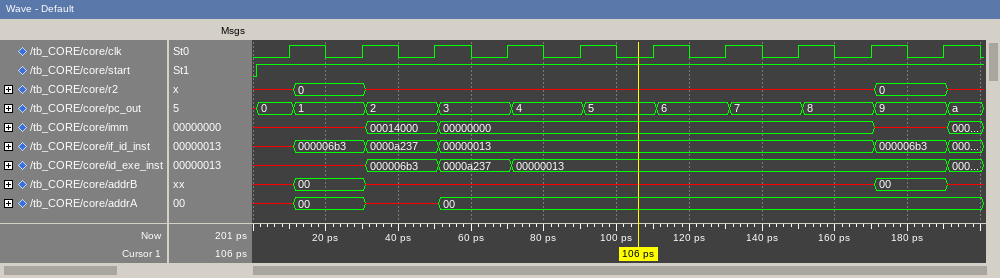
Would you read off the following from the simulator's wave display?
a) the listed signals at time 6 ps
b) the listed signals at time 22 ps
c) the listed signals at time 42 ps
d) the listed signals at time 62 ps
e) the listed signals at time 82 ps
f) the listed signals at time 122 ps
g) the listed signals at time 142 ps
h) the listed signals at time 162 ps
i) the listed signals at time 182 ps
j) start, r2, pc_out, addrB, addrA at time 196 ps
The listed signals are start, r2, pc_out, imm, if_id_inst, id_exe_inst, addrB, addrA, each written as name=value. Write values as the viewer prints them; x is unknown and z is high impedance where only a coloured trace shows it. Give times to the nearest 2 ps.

start=1, r2=x, pc_out=0, imm=x, if_id_inst=x, id_exe_inst=x, addrB=x, addrA=x
start=1, r2=0, pc_out=1, imm=x, if_id_inst=000006b3, id_exe_inst=x, addrB=00, addrA=00
start=1, r2=x, pc_out=2, imm=00014000, if_id_inst=0000a237, id_exe_inst=000006b3, addrB=x, addrA=x
start=1, r2=x, pc_out=3, imm=00000000, if_id_inst=00000013, id_exe_inst=0000a237, addrB=x, addrA=00
start=1, r2=x, pc_out=4, imm=00000000, if_id_inst=00000013, id_exe_inst=00000013, addrB=x, addrA=00
start=1, r2=x, pc_out=6, imm=00000000, if_id_inst=00000013, id_exe_inst=00000013, addrB=x, addrA=00
start=1, r2=x, pc_out=7, imm=00000000, if_id_inst=00000013, id_exe_inst=00000013, addrB=x, addrA=00
start=1, r2=x, pc_out=8, imm=00000000, if_id_inst=00000013, id_exe_inst=00000013, addrB=x, addrA=00
start=1, r2=0, pc_out=9, imm=x, if_id_inst=000006b3, id_exe_inst=00000013, addrB=00, addrA=00
start=1, r2=x, pc_out=a, addrB=x, addrA=00
